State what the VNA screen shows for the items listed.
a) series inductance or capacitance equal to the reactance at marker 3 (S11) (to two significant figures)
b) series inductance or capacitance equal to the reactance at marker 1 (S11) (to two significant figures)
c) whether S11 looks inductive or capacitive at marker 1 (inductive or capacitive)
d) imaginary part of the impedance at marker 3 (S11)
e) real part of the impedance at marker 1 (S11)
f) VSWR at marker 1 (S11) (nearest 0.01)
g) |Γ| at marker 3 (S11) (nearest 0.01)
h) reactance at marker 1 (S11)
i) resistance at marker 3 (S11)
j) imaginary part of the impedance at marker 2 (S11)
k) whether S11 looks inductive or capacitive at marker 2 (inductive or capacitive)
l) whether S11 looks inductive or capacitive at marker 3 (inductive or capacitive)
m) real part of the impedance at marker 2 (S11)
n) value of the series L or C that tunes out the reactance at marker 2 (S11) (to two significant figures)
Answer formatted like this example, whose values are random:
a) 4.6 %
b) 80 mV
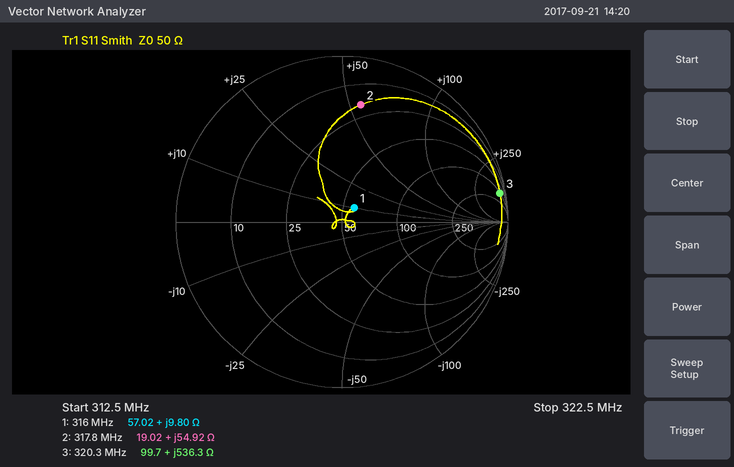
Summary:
a) 270 nH
b) 4.9 nH
c) inductive
d) +536.3 Ω
e) 57.02 Ω
f) 1.25
g) 0.97
h) +9.80 Ω
i) 99.7 Ω
j) +54.92 Ω
k) inductive
l) inductive
m) 19.02 Ω
n) 9.1 pF
